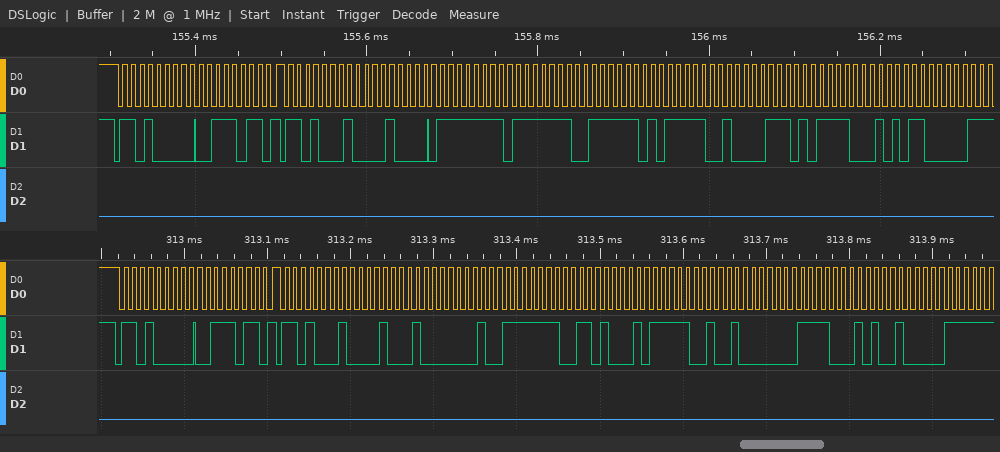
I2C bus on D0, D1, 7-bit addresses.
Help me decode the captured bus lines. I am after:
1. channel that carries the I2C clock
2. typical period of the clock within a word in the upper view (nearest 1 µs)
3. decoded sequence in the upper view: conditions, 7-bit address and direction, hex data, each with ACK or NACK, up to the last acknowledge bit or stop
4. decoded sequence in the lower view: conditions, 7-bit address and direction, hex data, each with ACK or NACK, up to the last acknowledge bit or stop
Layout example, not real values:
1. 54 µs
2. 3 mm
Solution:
1. D0
2. 10 µs
3. start, address 68 write ACK, 3B ACK, repeated start, address 68 read ACK, 10 ACK, FF ACK, FE ACK, FD ACK, F9 ACK, 1D ACK, F1 ACK, B0 ACK
4. start, address 68 write ACK, 3B ACK, repeated start, address 68 read ACK, 11 ACK, 02 ACK, FE ACK, D1 ACK, F9 ACK, 40 ACK, F1 ACK, 90 ACK
